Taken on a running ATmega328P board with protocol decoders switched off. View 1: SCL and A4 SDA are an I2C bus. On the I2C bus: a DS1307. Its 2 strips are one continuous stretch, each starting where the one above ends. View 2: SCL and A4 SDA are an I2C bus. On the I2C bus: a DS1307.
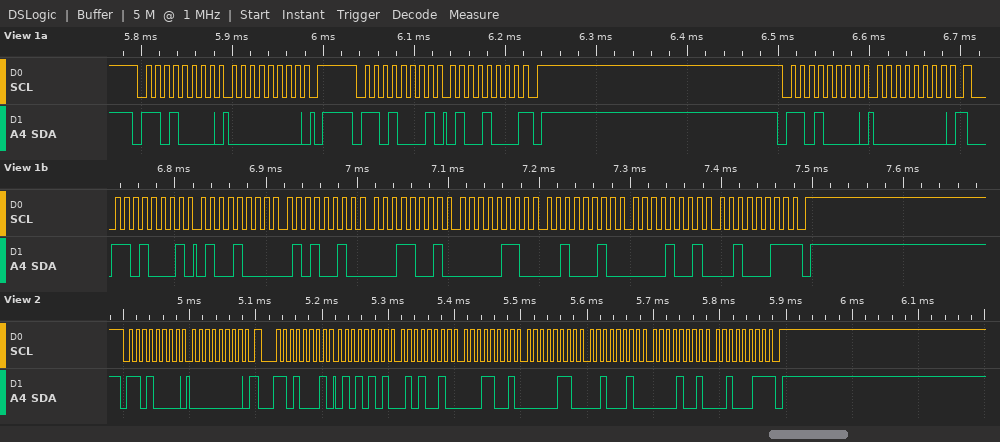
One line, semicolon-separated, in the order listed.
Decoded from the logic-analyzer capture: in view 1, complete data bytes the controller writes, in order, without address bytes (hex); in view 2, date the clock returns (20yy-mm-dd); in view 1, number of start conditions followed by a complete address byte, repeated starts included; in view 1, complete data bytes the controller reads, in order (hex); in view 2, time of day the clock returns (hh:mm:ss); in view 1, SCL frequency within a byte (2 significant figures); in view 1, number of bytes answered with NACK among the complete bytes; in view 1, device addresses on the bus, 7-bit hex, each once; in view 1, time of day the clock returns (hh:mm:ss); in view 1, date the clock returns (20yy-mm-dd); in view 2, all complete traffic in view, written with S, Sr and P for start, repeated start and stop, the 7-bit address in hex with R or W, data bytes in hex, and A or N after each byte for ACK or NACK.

00 00; 2023-09-22; 4; 48 48 52 19 06 22 09 23; 19:52:55; 100 kHz; 2; 0x68; 19:52:48; 2023-09-22; S 68W A 00 A Sr 68R A 55 A 52 A 19 A 06 A 22 A 09 A 23 N P
